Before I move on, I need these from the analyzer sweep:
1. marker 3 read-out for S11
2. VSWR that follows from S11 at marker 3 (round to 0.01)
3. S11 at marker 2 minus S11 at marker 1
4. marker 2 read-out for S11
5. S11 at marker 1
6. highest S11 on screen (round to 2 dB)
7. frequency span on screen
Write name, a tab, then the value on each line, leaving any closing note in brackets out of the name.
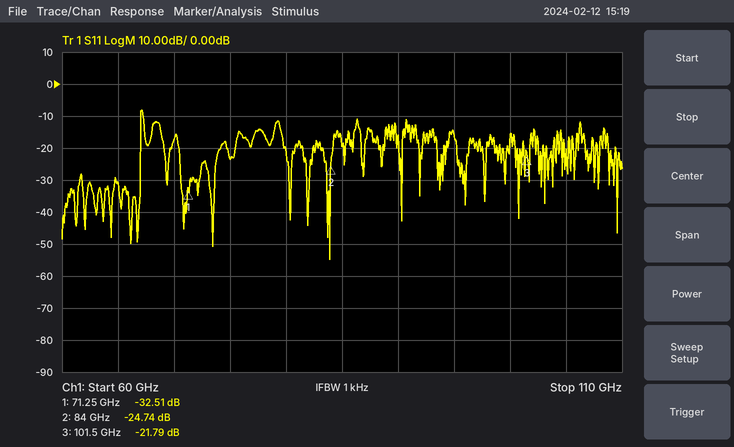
marker 3 read-out for S11	-21.79 dB
VSWR that follows from S11 at marker 3	1.18
S11 at marker 2 minus S11 at marker 1	7.77 dB
marker 2 read-out for S11	-24.74 dB
S11 at marker 1	-32.51 dB
highest S11 on screen	-8 dB
frequency span on screen	50 GHz
